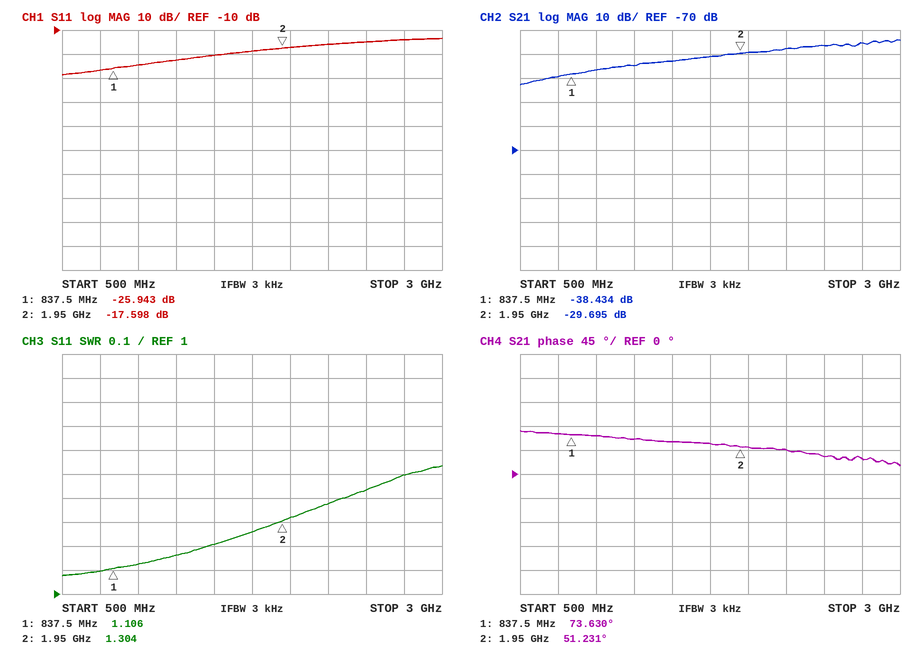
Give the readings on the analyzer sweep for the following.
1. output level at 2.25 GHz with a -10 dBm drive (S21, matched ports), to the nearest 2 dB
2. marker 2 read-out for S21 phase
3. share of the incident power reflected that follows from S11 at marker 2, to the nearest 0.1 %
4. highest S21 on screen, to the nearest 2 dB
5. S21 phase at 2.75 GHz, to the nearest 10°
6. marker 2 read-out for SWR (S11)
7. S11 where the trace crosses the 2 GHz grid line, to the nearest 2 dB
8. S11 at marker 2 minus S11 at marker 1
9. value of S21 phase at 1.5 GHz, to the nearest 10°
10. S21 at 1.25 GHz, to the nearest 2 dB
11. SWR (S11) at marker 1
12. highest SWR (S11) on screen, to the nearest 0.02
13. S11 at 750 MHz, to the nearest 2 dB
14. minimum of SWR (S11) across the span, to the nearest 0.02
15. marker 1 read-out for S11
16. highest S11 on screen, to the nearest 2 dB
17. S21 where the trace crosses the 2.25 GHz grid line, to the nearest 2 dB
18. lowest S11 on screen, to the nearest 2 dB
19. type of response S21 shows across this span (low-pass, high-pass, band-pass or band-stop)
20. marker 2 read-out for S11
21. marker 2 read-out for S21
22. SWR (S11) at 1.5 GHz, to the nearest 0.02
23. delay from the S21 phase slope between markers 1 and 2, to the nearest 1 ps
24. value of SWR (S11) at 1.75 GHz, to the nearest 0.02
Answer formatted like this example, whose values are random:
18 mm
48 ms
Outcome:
-38 dBm
51.231°
1.7 %
-24 dB
30°
1.304
-18 dB
8.345 dB
60°
-34 dB
1.106
1.54
-26 dB
1.08
-25.943 dB
-14 dB
-28 dB
-28 dB
high-pass
-17.598 dB
-29.695 dB
1.20
56 ps
1.26
